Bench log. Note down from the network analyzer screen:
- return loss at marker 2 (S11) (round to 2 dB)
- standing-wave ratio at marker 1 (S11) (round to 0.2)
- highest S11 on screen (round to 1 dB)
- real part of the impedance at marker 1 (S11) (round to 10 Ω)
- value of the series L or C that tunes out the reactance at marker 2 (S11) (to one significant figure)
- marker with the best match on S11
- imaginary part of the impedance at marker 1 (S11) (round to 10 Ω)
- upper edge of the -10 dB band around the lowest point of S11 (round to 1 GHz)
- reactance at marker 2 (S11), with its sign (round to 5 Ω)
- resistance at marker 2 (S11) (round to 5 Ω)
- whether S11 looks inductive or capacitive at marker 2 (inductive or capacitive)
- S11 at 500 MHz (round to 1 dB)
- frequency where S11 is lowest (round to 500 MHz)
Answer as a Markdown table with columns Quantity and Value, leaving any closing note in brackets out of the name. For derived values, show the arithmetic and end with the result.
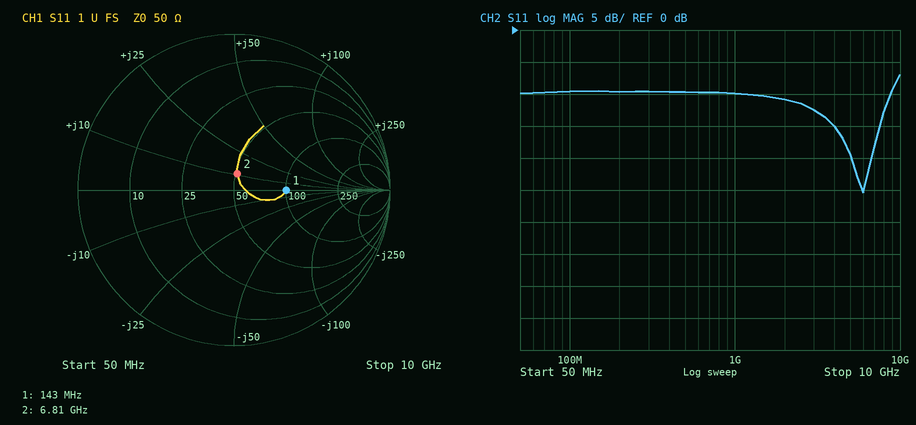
| Quantity | Value |
|---|---|
| return loss at marker 2 (S11) | 20 dB |
| standing-wave ratio at marker 1 (S11) | 2.0 |
| highest S11 on screen | -7 dB |
| real part of the impedance at marker 1 (S11) | 100 Ω |
| value of the series L or C that tunes out the reactance at marker 2 (S11) | C = 1/(2π × 6.81 GHz × 10 Ω) ≈ 2 pF |
| marker with the best match on S11 | marker 2 |
| imaginary part of the impedance at marker 1 (S11) | 0 Ω |
| upper edge of the -10 dB band around the lowest point of S11 | 9 GHz |
| reactance at marker 2 (S11), with its sign | +10 Ω |
| resistance at marker 2 (S11) | 50 Ω |
| whether S11 looks inductive or capacitive at marker 2 | inductive |
| S11 at 500 MHz | -10 dB |
| frequency where S11 is lowest | 6.0 GHz |
